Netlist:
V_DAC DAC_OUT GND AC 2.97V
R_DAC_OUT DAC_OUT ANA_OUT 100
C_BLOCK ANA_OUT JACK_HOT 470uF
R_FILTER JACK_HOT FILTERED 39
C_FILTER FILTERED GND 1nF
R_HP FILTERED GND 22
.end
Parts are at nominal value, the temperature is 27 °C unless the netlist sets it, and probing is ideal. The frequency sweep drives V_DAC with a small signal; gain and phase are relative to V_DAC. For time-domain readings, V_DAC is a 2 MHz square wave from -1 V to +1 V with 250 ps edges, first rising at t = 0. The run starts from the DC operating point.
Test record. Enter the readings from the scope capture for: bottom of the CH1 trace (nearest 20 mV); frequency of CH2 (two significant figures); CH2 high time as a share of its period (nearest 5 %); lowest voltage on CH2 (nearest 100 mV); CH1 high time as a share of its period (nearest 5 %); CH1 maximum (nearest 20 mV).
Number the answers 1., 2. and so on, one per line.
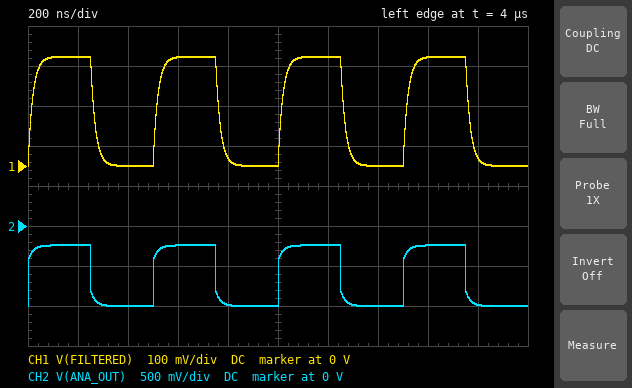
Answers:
1. 0 V
2. 2.0 MHz
3. 50 %
4. -1.0 V
5. 50 %
6. 280 mV
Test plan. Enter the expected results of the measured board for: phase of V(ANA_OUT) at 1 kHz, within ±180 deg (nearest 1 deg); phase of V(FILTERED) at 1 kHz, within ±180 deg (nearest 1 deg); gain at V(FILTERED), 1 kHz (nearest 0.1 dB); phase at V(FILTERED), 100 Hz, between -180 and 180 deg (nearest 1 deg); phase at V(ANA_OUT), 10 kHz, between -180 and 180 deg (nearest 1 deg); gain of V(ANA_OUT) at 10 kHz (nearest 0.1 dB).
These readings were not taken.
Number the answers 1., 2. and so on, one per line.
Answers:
1. 0 deg
2. 0 deg
3. -17.3 dB
4. 1 deg
5. 0 deg
6. -8.4 dB
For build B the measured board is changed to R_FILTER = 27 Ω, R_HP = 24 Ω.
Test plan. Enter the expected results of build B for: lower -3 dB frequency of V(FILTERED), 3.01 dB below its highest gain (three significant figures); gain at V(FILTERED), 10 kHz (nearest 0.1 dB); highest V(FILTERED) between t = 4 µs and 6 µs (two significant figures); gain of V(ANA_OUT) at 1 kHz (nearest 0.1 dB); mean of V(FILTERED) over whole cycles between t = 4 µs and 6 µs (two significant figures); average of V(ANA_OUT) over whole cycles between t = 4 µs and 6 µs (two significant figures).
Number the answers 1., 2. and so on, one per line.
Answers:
1. 2.24 Hz
2. -16.0 dB
3. 320 mV
4. -9.4 dB
5. 160 mV
6. -660 mV
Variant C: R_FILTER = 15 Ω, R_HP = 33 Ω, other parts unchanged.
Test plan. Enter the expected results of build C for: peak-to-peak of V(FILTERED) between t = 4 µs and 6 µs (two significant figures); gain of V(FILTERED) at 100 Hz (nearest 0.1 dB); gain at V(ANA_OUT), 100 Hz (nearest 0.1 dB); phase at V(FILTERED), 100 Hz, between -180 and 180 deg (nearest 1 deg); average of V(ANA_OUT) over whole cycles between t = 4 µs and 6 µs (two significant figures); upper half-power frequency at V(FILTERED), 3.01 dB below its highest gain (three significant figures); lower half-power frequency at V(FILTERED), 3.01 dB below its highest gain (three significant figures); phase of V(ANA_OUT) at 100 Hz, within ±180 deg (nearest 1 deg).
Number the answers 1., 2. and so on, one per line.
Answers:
1. 450 mV
2. -13.0 dB
3. -9.8 dB
4. 1 deg
5. -680 mV
6. 6.21 MHz
7. 2.29 Hz
8. -3 deg
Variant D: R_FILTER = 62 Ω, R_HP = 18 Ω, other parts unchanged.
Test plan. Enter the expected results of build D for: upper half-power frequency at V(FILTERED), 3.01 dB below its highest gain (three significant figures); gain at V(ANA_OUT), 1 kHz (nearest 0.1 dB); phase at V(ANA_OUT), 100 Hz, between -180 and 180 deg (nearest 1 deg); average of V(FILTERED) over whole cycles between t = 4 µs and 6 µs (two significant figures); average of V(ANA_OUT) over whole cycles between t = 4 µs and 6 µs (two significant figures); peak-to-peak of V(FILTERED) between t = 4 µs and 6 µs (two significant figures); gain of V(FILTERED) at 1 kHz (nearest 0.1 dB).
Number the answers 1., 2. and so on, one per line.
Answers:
1. 9.82 MHz
2. -7.0 dB
3. -1 deg
4. 100 mV
5. -560 mV
6. 200 mV
7. -20.0 dB
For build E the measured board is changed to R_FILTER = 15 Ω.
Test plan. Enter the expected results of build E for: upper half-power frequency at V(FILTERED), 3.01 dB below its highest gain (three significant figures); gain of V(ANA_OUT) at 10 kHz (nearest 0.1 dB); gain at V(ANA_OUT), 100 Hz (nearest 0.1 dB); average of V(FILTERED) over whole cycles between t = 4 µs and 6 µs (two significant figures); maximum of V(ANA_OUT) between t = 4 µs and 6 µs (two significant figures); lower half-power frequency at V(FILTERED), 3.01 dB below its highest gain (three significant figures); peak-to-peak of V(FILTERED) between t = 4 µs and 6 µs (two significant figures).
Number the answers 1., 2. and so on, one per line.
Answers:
1. 8.62 MHz
2. -11.4 dB
3. -11.3 dB
4. 160 mV
5. -460 mV
6. 2.47 Hz
7. 320 mV
